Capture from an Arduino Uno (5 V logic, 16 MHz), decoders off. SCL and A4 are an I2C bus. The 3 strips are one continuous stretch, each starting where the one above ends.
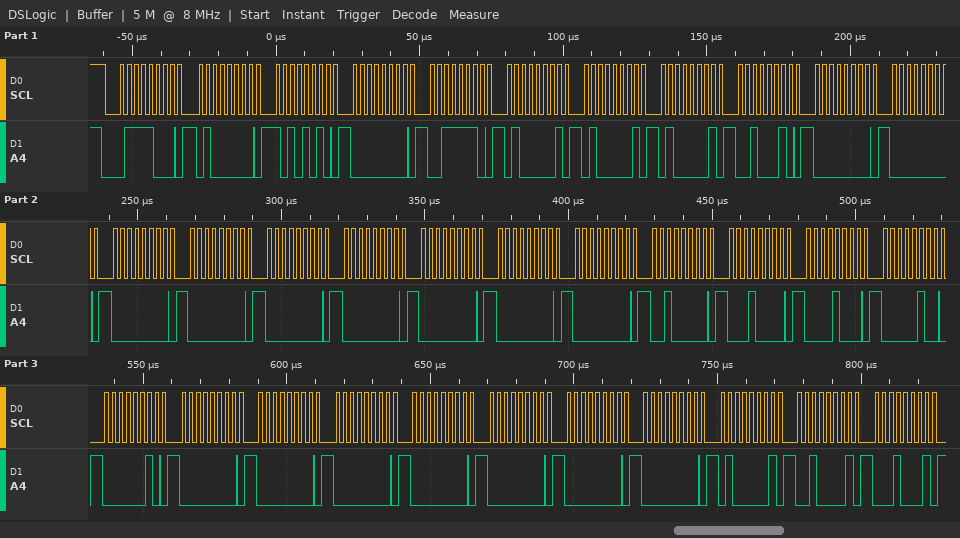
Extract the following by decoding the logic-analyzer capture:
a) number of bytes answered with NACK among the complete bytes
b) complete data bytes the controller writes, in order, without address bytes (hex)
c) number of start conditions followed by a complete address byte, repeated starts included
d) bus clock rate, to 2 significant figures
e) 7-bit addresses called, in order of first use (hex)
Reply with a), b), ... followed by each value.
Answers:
a) 0
b) 40 AA 00 3E 41 41 41 22 00 00 00 00 00 00 00 00 00 20 10 08 04 02 00 00 00 00 00 00 00 41 21 11
c) 1
d) 400 kHz
e) 0x3C
